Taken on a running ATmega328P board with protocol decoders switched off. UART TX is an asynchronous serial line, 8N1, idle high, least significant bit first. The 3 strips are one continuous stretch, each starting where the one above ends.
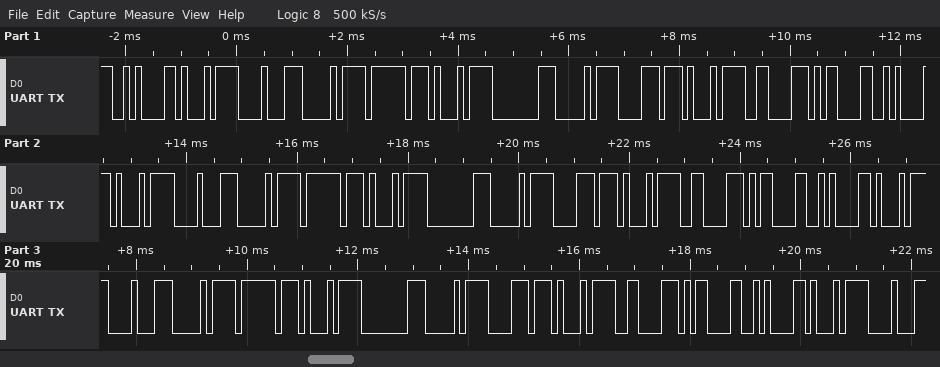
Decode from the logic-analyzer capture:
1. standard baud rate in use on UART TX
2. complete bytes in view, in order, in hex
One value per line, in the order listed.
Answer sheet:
9600 baud
0A D1 88 D0 BF D1 80 D0 B8 D1 86 0D 0A D1 88 D0 BF D1 80 D0 B8 D1 86 0D 0A D1 88 D0 BF D1 80 D0 B8 D1 86 0D 0A D1 88
